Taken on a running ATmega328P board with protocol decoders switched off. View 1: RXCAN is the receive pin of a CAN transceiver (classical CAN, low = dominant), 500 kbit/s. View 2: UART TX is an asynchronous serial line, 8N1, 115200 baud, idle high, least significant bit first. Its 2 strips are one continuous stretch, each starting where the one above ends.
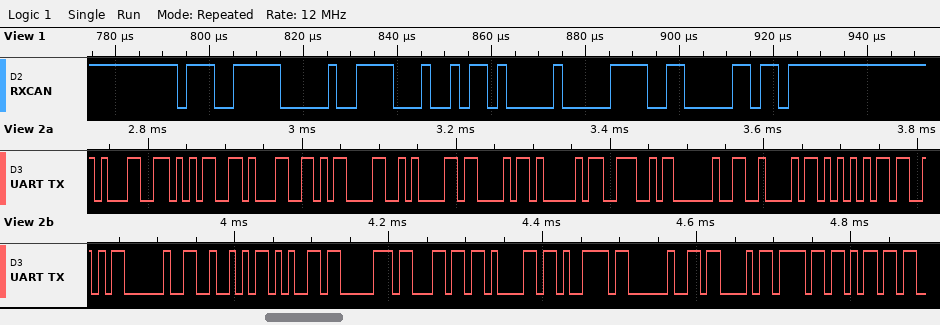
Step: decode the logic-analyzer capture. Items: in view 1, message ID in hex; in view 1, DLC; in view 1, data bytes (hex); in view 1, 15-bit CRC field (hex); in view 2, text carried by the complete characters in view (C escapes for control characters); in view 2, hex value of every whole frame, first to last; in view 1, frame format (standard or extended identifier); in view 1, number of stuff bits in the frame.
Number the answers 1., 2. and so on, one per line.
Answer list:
1. 0x73E
2. 3
3. C4 B4 00
4. 0x7305
5. "151\r\nCAN BUS Replay Com"
6. 0x31 0x35 0x31 0x0D 0x0A 0x43 0x41 0x4E 0x20 0x42 0x55 0x53 0x20 0x52 0x65 0x70 0x6C 0x61 0x79 0x20 0x43 0x6F 0x6D
7. standard
8. 5
